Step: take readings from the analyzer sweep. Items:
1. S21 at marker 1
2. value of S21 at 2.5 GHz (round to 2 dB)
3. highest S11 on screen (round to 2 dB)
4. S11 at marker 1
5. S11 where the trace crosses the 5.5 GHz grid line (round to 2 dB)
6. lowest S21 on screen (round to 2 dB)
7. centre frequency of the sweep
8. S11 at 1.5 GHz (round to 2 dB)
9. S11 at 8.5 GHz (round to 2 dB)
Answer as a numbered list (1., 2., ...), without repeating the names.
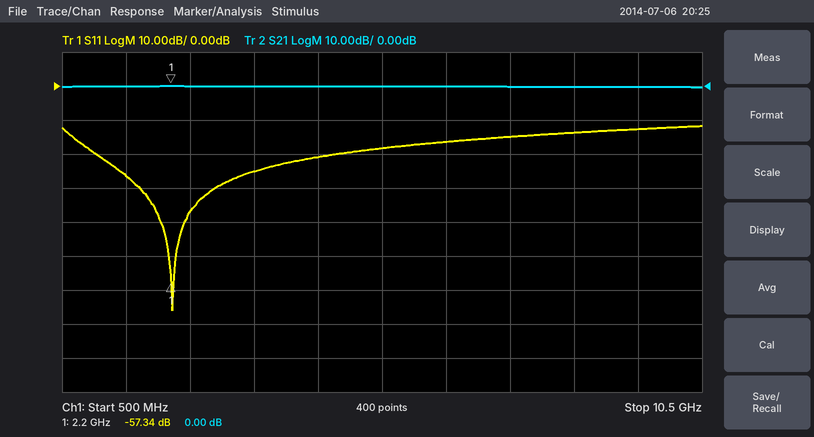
1. 0.00 dB
2. 0 dB
3. -12 dB
4. -57.34 dB
5. -18 dB
6. 0 dB
7. 5.5 GHz
8. -26 dB
9. -14 dB
